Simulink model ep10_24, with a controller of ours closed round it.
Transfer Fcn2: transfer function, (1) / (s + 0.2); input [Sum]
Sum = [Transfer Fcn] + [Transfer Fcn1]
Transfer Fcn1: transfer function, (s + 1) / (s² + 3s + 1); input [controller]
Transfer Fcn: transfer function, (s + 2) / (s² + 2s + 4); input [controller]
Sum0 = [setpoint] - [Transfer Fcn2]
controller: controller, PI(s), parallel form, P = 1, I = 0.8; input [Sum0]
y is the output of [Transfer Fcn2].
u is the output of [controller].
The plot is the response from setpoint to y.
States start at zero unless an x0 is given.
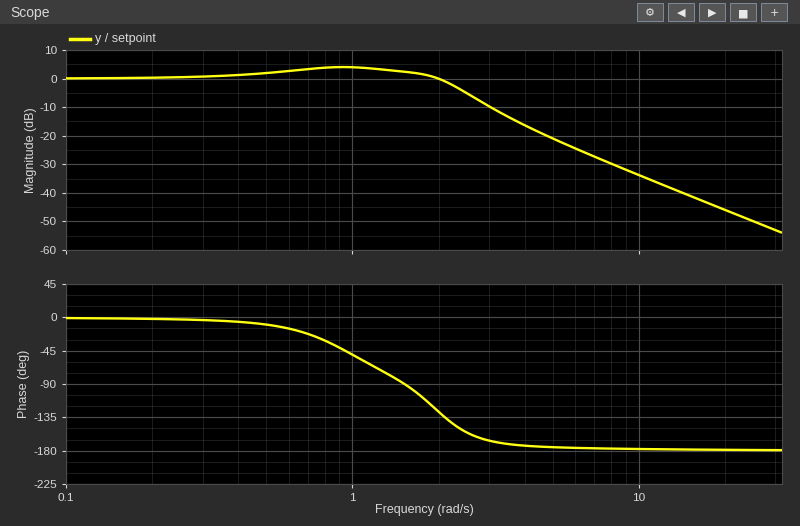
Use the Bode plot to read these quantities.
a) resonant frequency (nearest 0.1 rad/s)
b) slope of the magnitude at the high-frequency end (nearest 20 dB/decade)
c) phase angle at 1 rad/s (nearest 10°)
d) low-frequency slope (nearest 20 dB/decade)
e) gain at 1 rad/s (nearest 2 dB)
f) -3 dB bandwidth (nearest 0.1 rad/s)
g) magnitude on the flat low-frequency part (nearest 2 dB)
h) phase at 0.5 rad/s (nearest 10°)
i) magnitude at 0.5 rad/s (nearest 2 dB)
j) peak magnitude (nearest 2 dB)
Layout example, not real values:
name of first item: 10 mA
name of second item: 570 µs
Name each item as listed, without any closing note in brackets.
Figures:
resonant frequency: 0.9 rad/s
slope of the magnitude at the high-frequency end: -40 dB/decade
phase angle at 1 rad/s: -50°
low-frequency slope: 0 dB/decade
gain at 1 rad/s: 4 dB
-3 dB bandwidth: 2.3 rad/s
magnitude on the flat low-frequency part: 0 dB
phase at 0.5 rad/s: -10°
magnitude at 0.5 rad/s: 2 dB
peak magnitude: 4 dB
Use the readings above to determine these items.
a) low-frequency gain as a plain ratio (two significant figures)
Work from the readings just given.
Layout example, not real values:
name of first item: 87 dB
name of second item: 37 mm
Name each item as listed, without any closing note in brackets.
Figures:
low-frequency gain as a plain ratio: 1.0
